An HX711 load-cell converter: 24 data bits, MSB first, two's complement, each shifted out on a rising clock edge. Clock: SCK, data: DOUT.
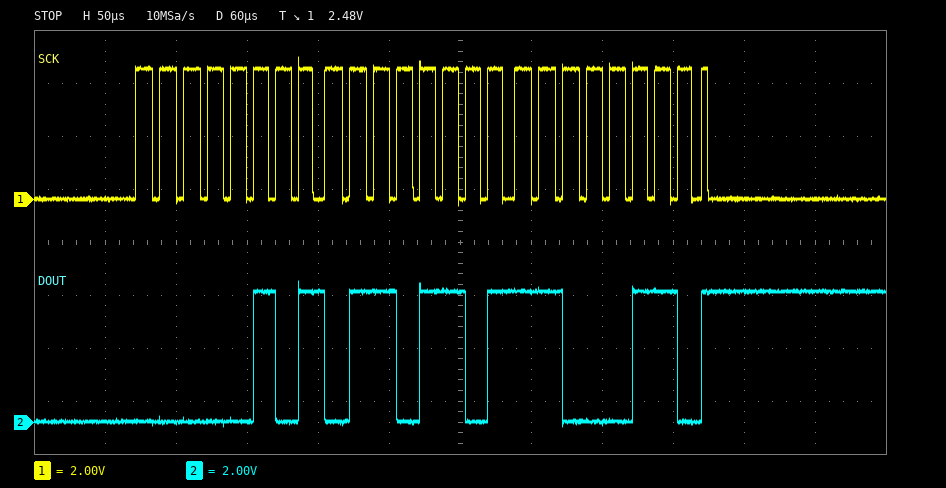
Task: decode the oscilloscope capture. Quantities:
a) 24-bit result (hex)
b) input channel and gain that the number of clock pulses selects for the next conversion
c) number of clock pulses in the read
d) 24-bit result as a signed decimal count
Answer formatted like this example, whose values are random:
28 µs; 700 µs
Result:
0x056DC6; channel A, gain 128; 25; 355782
